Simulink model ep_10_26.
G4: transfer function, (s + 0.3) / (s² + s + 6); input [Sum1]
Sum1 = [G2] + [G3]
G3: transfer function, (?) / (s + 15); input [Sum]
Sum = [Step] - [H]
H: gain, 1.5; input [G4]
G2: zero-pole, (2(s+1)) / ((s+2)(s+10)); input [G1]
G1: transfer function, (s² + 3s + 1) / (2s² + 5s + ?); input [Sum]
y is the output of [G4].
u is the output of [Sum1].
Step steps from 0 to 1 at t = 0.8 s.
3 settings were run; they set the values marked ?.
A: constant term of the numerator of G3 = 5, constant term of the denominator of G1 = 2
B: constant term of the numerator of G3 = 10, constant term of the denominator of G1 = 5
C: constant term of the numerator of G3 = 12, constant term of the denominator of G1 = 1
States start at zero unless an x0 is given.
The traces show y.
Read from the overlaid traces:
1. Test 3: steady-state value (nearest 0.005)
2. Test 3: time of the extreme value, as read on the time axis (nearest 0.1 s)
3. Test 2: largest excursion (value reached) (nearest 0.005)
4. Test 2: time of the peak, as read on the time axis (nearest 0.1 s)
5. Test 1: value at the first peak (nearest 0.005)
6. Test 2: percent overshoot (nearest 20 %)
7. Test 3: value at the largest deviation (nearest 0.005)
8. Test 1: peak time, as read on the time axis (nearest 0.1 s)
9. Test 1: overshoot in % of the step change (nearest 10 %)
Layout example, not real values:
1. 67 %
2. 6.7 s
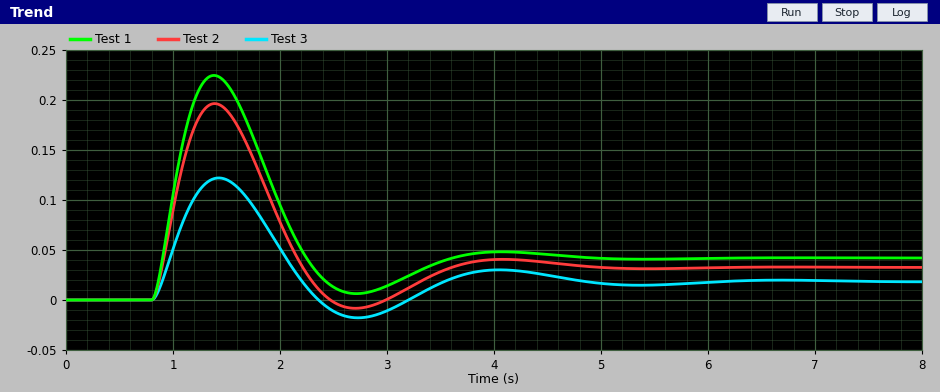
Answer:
1. 0.020
2. 1.4 s
3. 0.195
4. 1.4 s
5. 0.225
6. 500 %
7. 0.120
8. 1.4 s
9. 430 %
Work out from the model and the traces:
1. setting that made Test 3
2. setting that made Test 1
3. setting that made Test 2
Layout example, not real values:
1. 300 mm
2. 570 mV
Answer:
1. A
2. C
3. B
